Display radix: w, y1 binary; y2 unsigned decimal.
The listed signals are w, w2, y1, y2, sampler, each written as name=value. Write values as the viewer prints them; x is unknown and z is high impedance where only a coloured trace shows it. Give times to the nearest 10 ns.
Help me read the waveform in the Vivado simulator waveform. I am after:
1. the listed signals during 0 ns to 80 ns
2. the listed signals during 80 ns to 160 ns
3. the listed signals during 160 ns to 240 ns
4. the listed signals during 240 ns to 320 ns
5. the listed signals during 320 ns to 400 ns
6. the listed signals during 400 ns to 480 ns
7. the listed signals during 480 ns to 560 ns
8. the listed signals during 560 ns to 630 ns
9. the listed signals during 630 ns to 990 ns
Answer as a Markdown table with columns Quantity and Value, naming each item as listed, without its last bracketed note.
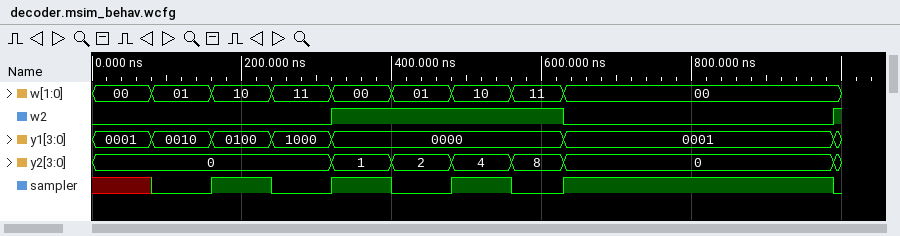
| Quantity | Value |
|---|---|
| the listed signals during 0 ns to 80 ns | w=00, w2=0, y1=0001, y2=0, sampler=x |
| the listed signals during 80 ns to 160 ns | w=01, w2=0, y1=0010, y2=0, sampler=0 |
| the listed signals during 160 ns to 240 ns | w=10, w2=0, y1=0100, y2=0, sampler=1 |
| the listed signals during 240 ns to 320 ns | w=11, w2=0, y1=1000, y2=0, sampler=0 |
| the listed signals during 320 ns to 400 ns | w=00, w2=1, y1=0000, y2=1, sampler=1 |
| the listed signals during 400 ns to 480 ns | w=01, w2=1, y1=0000, y2=2, sampler=0 |
| the listed signals during 480 ns to 560 ns | w=10, w2=1, y1=0000, y2=4, sampler=1 |
| the listed signals during 560 ns to 630 ns | w=11, w2=1, y1=0000, y2=8, sampler=0 |
| the listed signals during 630 ns to 990 ns | w=00, w2=0, y1=0001, y2=0, sampler=1 |
